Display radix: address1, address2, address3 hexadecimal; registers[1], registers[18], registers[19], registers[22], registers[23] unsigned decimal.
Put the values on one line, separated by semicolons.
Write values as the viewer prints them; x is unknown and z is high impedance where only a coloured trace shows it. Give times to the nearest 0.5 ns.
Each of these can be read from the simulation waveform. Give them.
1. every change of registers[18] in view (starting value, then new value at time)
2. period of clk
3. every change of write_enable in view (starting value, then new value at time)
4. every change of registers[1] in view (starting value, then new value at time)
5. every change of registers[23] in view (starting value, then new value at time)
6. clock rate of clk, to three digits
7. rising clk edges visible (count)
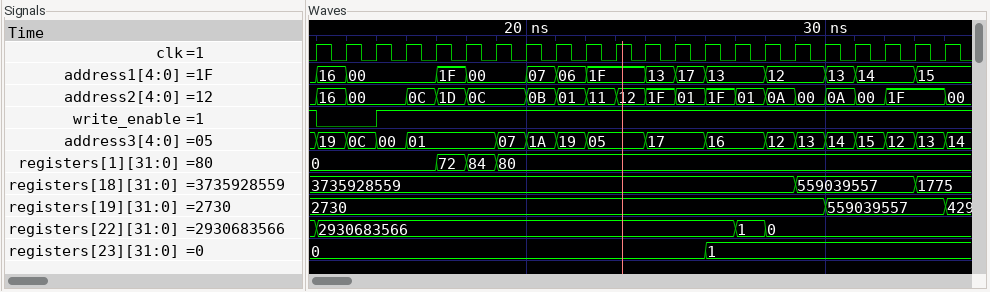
3735928559, 559039557 at 29 ns, 1775 at 33 ns; 1 ns; 1, 0 at 13 ns, 1 at 15 ns; 0, 72 at 17 ns, 84 at 18 ns, 80 at 19 ns; 0, 1 at 26 ns; 1.00 GHz; 22
